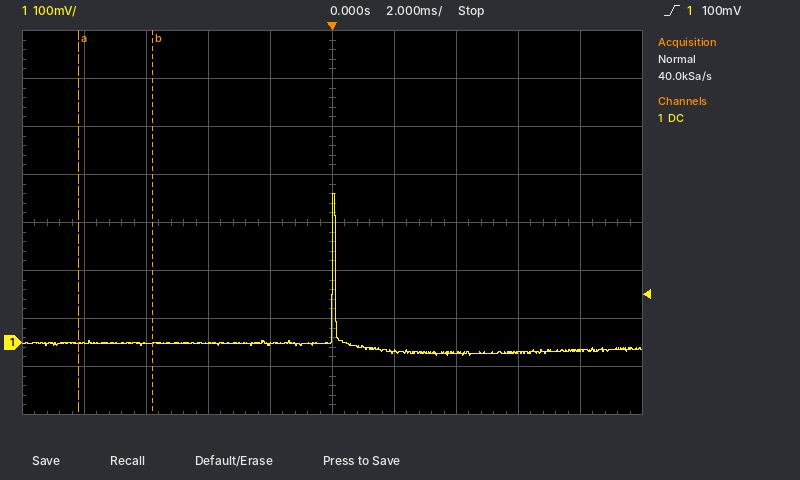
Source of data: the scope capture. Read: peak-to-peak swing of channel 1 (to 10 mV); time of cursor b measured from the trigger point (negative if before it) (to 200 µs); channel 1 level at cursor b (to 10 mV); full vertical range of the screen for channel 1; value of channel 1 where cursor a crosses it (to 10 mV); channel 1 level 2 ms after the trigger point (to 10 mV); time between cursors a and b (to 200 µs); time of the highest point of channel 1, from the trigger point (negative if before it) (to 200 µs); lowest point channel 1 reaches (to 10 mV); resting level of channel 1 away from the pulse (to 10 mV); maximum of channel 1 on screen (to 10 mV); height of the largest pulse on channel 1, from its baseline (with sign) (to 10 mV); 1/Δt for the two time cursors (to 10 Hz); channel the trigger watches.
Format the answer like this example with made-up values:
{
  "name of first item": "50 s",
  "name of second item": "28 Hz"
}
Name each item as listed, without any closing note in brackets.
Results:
{
  "peak-to-peak swing of channel 1": "340 mV",
  "time of cursor b measured from the trigger point (negative if before it)": "-5.8 ms",
  "channel 1 level at cursor b": "0 mV",
  "full vertical range of the screen for channel 1": "800 mV",
  "value of channel 1 where cursor a crosses it": "0 mV",
  "channel 1 level 2 ms after the trigger point": "-20 mV",
  "time between cursors a and b": "2.4 ms",
  "time of the highest point of channel 1, from the trigger point (negative if before it)": "0.0 ms",
  "lowest point channel 1 reaches": "-30 mV",
  "resting level of channel 1 away from the pulse": "0 mV",
  "maximum of channel 1 on screen": "310 mV",
  "height of the largest pulse on channel 1, from its baseline (with sign)": "+310 mV",
  "1/Δt for the two time cursors": "420 Hz",
  "channel the trigger watches": "channel 1"
}
